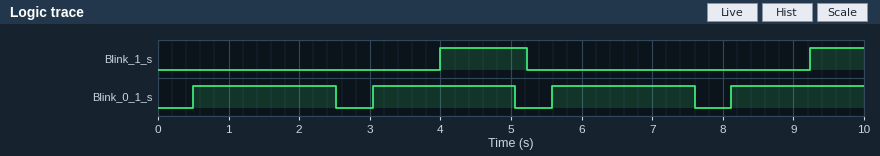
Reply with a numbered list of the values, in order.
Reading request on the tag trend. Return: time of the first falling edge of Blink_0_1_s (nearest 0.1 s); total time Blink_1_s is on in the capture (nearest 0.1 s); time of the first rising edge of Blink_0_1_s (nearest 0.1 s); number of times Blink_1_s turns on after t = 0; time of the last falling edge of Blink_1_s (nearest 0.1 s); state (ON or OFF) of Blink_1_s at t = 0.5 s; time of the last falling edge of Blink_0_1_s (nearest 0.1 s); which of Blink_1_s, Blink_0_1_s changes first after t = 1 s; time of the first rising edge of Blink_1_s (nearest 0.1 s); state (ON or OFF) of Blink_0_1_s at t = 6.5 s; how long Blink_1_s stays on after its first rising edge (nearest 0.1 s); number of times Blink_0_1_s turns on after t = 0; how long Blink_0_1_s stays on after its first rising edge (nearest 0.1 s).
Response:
1. 2.5 s
2. 2.0 s
3. 0.5 s
4. 2
5. 5.2 s
6. OFF
7. 7.6 s
8. Blink_0_1_s
9. 4.0 s
10. ON
11. 1.2 s
12. 4
13. 2.0 s
